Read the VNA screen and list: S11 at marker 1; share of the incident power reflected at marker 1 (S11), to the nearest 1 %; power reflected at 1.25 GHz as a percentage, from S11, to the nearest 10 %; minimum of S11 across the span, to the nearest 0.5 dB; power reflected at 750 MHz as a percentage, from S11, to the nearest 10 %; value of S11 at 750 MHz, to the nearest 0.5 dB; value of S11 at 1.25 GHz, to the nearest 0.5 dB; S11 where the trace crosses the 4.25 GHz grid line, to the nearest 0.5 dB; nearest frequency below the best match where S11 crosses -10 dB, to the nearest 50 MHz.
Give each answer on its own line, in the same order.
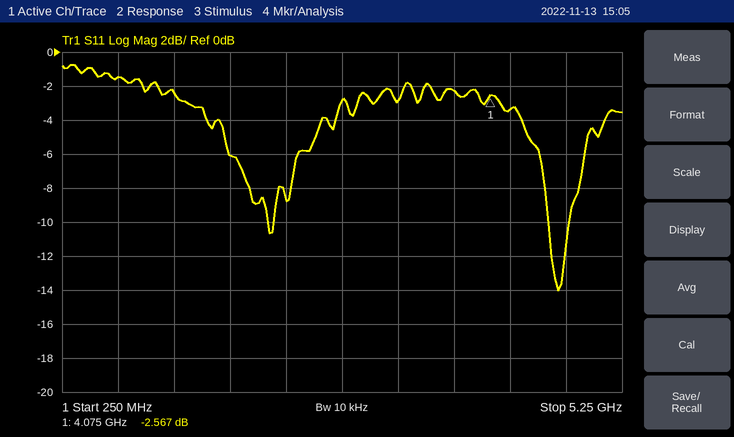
-2.567 dB
55 %
60 %
-14.0 dB
70 %
-1.5 dB
-2.5 dB
-3.5 dB
4.60 GHz
